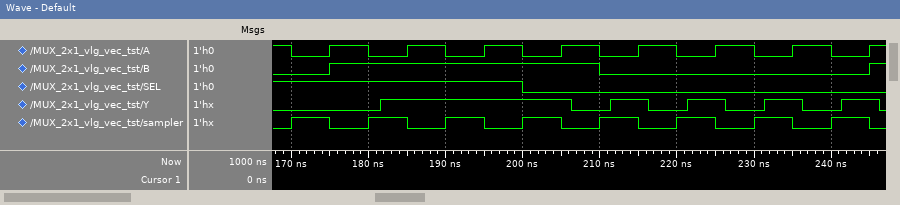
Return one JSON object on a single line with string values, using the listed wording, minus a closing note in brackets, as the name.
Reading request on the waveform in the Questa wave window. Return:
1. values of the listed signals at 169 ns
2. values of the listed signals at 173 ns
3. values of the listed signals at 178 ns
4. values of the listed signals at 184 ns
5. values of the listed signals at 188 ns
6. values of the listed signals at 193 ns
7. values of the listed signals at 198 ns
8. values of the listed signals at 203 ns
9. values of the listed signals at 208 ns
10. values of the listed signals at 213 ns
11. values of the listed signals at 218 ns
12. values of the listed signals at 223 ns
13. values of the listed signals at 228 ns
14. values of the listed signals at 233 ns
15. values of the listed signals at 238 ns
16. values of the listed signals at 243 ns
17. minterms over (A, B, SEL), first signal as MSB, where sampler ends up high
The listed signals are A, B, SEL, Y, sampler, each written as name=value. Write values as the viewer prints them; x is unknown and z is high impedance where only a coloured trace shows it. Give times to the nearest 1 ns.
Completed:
{"values of the listed signals at 169 ns": "A=1, B=0, SEL=1, Y=0, sampler=0", "values of the listed signals at 173 ns": "A=0, B=0, SEL=1, Y=0, sampler=1", "values of the listed signals at 178 ns": "A=1, B=1, SEL=1, Y=0, sampler=0", "values of the listed signals at 184 ns": "A=0, B=1, SEL=1, Y=1, sampler=1", "values of the listed signals at 188 ns": "A=1, B=1, SEL=1, Y=1, sampler=0", "values of the listed signals at 193 ns": "A=0, B=1, SEL=1, Y=1, sampler=1", "values of the listed signals at 198 ns": "A=1, B=1, SEL=1, Y=1, sampler=0", "values of the listed signals at 203 ns": "A=0, B=1, SEL=0, Y=1, sampler=1", "values of the listed signals at 208 ns": "A=1, B=1, SEL=0, Y=0, sampler=0", "values of the listed signals at 213 ns": "A=0, B=0, SEL=0, Y=1, sampler=1", "values of the listed signals at 218 ns": "A=1, B=0, SEL=0, Y=0, sampler=0", "values of the listed signals at 223 ns": "A=0, B=0, SEL=0, Y=1, sampler=1", "values of the listed signals at 228 ns": "A=1, B=0, SEL=0, Y=0, sampler=0", "values of the listed signals at 233 ns": "A=0, B=0, SEL=0, Y=1, sampler=1", "values of the listed signals at 238 ns": "A=1, B=0, SEL=0, Y=0, sampler=0", "values of the listed signals at 243 ns": "A=0, B=0, SEL=0, Y=1, sampler=1", "minterms over (A, B, SEL), first signal as MSB, where sampler ends up high": "0, 1, 2, 3"}
